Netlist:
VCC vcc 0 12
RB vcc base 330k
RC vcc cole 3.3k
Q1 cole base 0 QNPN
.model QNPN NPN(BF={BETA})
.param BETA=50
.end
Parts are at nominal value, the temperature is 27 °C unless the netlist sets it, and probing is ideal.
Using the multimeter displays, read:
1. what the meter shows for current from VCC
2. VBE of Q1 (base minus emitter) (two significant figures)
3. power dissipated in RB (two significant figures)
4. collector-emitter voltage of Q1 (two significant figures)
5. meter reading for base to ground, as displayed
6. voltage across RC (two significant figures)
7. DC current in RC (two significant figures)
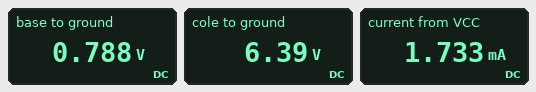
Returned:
1.733 mA
790 mV
380 µW
6.4 V
0.788 V
5.6 V
1.7 mA
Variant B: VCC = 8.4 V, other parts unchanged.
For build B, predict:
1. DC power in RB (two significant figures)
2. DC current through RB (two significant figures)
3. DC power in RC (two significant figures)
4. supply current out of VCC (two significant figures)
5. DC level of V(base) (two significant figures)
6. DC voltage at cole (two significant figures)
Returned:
180 µW
23 µA
4.4 mW
1.2 mA
780 mV
4.6 V
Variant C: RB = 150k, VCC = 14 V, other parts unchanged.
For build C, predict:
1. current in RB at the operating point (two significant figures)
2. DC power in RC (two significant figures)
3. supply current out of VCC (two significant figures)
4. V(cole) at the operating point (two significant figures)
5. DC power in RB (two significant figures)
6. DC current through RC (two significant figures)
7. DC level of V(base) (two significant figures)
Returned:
88 µA
58 mW
4.3 mA
180 mV
1.2 mW
4.2 mA
810 mV
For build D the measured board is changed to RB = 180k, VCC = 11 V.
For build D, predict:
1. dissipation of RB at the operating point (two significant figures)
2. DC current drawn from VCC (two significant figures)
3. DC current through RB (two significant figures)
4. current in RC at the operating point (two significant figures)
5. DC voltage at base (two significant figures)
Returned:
580 µW
2.9 mA
57 µA
2.8 mA
800 mV
